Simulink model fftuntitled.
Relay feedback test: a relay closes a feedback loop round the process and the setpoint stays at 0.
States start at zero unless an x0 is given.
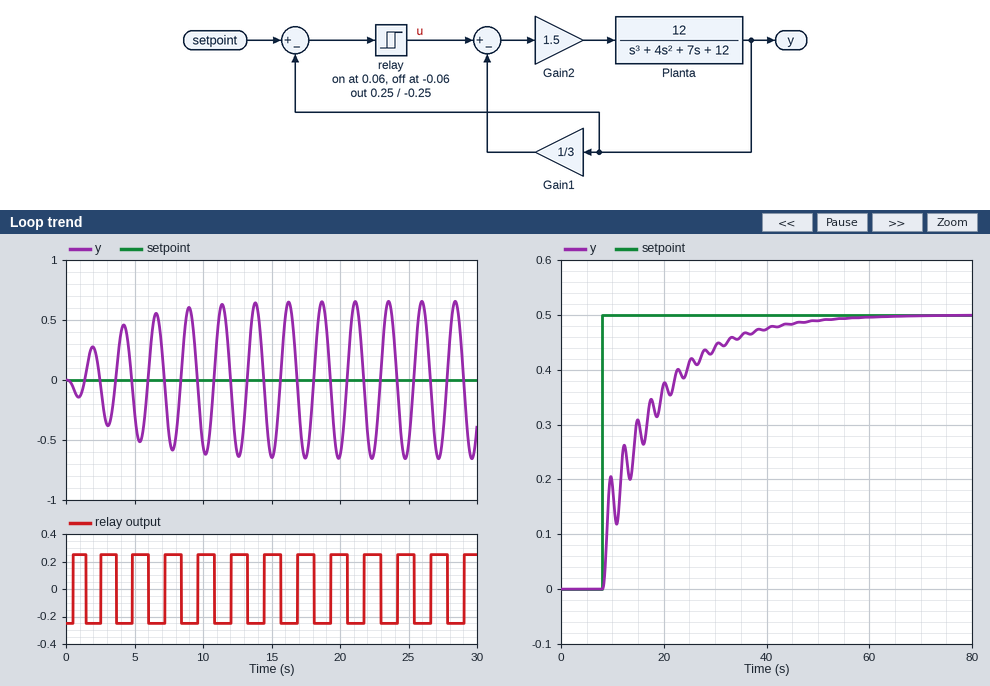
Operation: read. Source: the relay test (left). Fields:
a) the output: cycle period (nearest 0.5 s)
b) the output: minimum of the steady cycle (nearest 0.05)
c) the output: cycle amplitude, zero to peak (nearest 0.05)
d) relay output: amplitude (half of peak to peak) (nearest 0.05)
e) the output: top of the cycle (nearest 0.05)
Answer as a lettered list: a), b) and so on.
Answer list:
a) 2.5 s
b) -0.65
c) 0.65
d) 0.25
e) 0.65
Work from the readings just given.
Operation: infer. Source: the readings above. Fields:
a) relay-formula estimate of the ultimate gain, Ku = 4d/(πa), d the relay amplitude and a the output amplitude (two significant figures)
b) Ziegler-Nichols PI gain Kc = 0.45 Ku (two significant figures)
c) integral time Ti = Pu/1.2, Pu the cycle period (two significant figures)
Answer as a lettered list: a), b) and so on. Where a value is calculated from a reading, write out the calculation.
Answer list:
a) 4 × 0.25 / (π × 0.65) = 0.49
b) 0.45 × 0.49 = 0.22
c) 2.5 / 1.2 = 2.1 s
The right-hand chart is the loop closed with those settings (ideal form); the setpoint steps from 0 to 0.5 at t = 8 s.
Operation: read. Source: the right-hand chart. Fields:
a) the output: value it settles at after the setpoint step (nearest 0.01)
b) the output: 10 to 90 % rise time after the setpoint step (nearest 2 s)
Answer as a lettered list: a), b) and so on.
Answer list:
a) 0.50
b) 24 s
